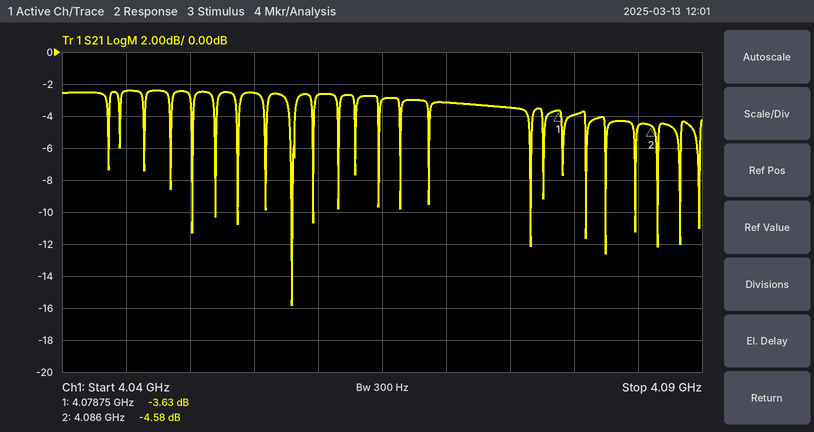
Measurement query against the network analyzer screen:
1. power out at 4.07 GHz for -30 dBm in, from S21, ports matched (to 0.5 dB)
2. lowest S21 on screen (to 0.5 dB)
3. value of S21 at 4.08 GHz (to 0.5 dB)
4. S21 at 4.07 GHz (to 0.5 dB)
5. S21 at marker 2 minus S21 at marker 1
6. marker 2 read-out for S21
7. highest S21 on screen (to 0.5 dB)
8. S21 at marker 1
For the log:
-33.0 dBm
-16.0 dB
-4.0 dB
-3.0 dB
-0.95 dB
-4.58 dB
-2.5 dB
-3.63 dB
